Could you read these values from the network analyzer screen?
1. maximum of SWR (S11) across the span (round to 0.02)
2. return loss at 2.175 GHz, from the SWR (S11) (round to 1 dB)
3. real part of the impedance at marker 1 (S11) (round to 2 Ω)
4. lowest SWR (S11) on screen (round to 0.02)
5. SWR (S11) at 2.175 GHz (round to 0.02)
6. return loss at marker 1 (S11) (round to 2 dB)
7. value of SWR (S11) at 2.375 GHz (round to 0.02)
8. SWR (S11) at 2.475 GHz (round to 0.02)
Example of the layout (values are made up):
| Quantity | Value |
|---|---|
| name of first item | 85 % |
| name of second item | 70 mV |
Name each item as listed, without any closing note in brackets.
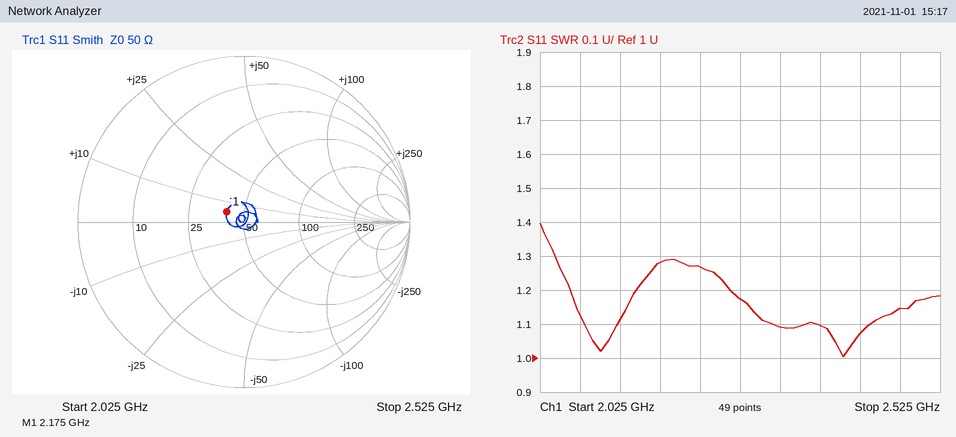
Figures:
| Quantity | Value |
|---|---|
| maximum of SWR (S11) across the span | 1.40 |
| return loss at 2.175 GHz, from the SWR (S11) | 18 dB |
| real part of the impedance at marker 1 (S11) | 40 Ω |
| lowest SWR (S11) on screen | 1.00 |
| SWR (S11) at 2.175 GHz | 1.28 |
| return loss at marker 1 (S11) | 18 dB |
| value of SWR (S11) at 2.375 GHz | 1.10 |
| SWR (S11) at 2.475 GHz | 1.14 |
